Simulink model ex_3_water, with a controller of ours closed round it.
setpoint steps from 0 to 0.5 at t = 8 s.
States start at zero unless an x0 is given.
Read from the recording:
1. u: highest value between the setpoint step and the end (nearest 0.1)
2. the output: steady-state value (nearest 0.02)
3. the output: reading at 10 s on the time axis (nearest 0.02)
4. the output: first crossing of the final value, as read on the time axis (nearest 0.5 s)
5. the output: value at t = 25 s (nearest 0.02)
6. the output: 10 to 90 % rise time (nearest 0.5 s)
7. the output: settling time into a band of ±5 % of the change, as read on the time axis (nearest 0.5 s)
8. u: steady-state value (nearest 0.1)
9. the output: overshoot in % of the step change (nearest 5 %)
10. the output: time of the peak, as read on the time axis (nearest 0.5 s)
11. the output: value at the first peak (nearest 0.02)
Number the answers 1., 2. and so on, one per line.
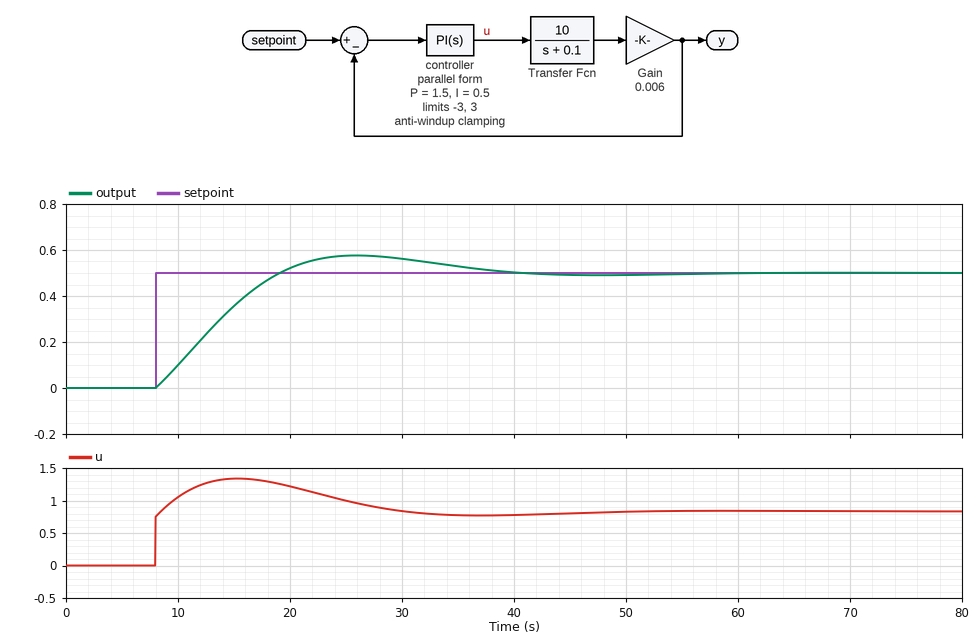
1. 1.3
2. 0.50
3. 0.10
4. 19.0 s
5. 0.58
6. 8.5 s
7. 35.5 s
8. 0.8
9. 15 %
10. 26.0 s
11. 0.58
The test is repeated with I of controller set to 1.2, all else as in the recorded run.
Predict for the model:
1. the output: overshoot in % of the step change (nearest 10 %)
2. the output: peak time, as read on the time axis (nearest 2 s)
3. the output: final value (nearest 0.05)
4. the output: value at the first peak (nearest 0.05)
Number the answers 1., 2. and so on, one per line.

1. 30 %
2. 20 s
3. 0.50
4. 0.65
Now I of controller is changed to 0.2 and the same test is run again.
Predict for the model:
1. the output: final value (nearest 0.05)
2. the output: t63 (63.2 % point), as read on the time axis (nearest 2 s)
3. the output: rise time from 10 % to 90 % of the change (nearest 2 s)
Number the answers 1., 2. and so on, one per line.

1. 0.50
2. 18 s
3. 18 s
